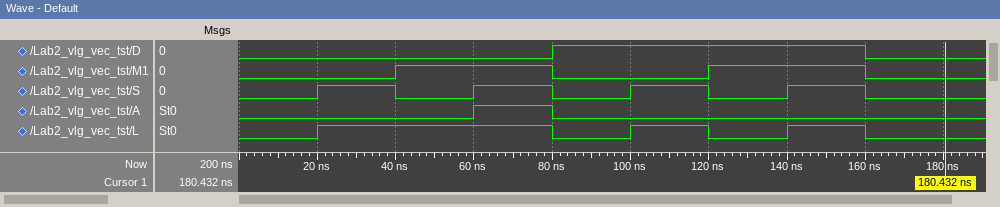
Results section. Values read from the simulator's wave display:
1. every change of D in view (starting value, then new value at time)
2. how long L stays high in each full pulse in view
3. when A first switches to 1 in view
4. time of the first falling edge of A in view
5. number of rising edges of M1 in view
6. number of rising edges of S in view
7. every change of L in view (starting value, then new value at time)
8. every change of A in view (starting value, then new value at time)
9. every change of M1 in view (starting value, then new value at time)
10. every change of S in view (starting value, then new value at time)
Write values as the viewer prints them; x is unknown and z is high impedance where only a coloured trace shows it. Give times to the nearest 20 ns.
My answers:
0, 1 at 80 ns, 0 at 160 ns
60 ns, 20 ns, 20 ns
60 ns
80 ns
2
4
0, 1 at 20 ns, 0 at 80 ns, 1 at 100 ns, 0 at 120 ns, 1 at 140 ns, 0 at 160 ns
0, 1 at 60 ns, 0 at 80 ns
0, 1 at 40 ns, 0 at 80 ns, 1 at 120 ns, 0 at 160 ns
0, 1 at 20 ns, 0 at 40 ns, 1 at 60 ns, 0 at 80 ns, 1 at 100 ns, 0 at 120 ns, 1 at 140 ns, 0 at 160 ns
